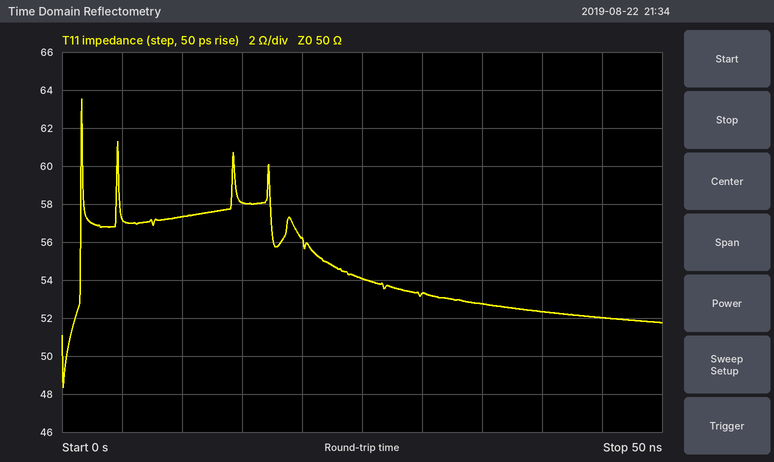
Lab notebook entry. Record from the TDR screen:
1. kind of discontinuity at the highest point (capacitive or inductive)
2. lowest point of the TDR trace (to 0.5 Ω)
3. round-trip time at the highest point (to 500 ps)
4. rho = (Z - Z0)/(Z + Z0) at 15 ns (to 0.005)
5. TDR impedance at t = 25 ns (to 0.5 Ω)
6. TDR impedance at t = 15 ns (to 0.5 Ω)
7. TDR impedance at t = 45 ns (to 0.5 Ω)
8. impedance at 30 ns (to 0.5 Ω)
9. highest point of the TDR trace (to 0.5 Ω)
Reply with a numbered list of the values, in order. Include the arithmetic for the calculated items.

1. inductive
2. 48.5 Ω
3. 1.5 ns
4. (58 − 50)/(58 + 50) ≈ +0.0741, so +0.075 to the nearest 0.005
5. 54.0 Ω
6. 58.0 Ω
7. 52.0 Ω
8. 53.5 Ω
9. 63.5 Ω
